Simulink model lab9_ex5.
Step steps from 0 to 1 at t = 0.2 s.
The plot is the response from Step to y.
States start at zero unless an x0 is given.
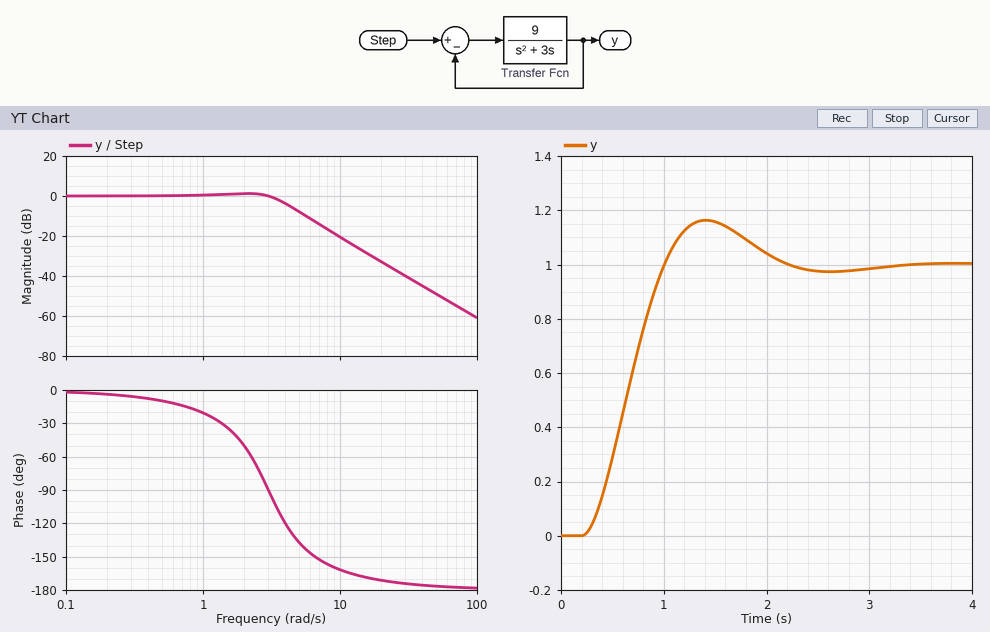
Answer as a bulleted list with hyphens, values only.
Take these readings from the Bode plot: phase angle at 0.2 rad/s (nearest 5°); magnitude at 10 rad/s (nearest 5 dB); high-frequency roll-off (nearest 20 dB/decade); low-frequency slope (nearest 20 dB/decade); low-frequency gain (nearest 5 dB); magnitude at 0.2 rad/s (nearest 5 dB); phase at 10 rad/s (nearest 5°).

- -5°
- -20 dB
- -40 dB/decade
- 0 dB/decade
- 0 dB
- 0 dB
- -160°
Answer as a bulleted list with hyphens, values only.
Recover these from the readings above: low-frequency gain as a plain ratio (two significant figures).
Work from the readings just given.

- 1.0
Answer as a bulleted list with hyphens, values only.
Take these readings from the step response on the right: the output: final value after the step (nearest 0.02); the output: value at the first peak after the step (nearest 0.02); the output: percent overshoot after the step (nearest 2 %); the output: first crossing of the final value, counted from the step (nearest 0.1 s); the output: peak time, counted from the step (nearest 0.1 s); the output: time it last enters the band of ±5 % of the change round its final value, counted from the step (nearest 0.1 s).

- 1.00
- 1.16
- 16 %
- 0.8 s
- 1.2 s
- 1.8 s
